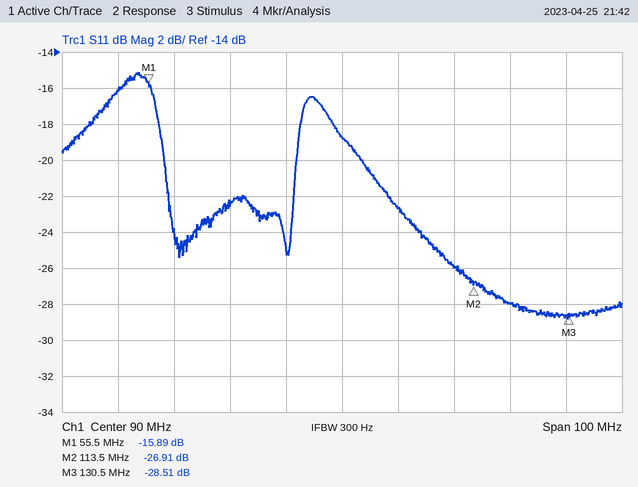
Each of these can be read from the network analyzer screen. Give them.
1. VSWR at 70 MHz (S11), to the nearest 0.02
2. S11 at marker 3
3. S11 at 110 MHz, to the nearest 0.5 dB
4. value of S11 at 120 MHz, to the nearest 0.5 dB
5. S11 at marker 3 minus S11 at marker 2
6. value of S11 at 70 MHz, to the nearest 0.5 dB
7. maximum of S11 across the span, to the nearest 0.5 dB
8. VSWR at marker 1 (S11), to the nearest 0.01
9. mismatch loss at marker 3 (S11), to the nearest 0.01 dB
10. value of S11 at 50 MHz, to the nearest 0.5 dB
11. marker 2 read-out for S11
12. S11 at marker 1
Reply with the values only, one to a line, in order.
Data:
1.16
-28.51 dB
-26.0 dB
-28.0 dB
-1.60 dB
-22.5 dB
-15.0 dB
1.38
0.01 dB
-16.0 dB
-26.91 dB
-15.89 dB
